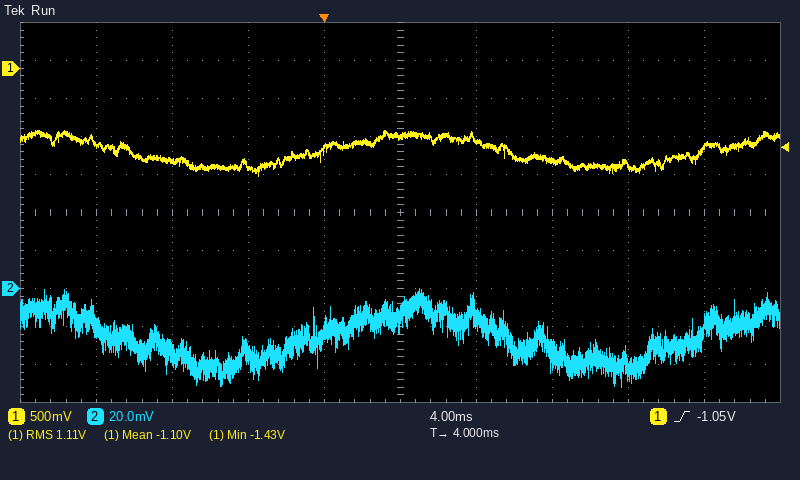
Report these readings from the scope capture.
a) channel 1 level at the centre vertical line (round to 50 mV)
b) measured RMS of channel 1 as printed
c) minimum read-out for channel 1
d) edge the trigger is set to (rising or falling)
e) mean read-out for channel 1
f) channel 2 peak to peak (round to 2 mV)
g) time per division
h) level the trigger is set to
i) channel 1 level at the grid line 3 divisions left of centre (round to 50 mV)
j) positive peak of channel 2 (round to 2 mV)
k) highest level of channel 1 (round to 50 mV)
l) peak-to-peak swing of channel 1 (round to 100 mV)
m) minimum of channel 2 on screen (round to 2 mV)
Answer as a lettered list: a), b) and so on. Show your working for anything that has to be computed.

a) -900 mV
b) 1.11 V
c) -1.43 V
d) rising
e) -1.10 V
f) 0 mV − (-52 mV) = 52 mV
g) 4 ms
h) -1.05 V
i) -1.20 V
j) 0 mV
k) -800 mV
l) 600 mV
m) -52 mV
